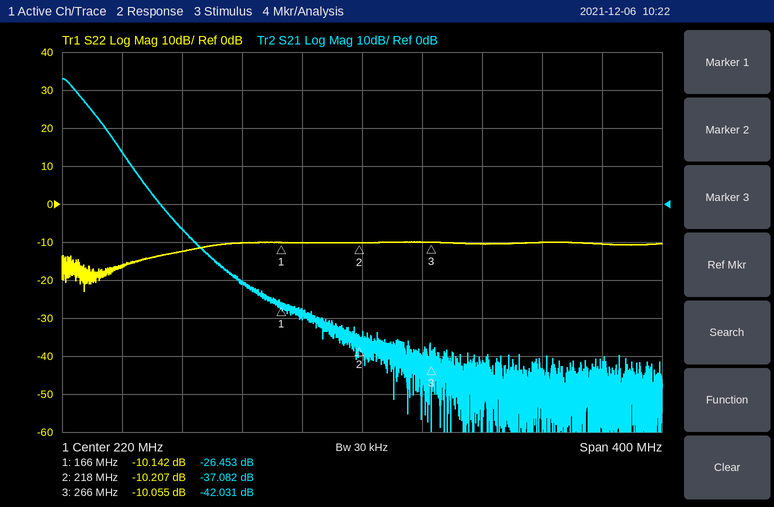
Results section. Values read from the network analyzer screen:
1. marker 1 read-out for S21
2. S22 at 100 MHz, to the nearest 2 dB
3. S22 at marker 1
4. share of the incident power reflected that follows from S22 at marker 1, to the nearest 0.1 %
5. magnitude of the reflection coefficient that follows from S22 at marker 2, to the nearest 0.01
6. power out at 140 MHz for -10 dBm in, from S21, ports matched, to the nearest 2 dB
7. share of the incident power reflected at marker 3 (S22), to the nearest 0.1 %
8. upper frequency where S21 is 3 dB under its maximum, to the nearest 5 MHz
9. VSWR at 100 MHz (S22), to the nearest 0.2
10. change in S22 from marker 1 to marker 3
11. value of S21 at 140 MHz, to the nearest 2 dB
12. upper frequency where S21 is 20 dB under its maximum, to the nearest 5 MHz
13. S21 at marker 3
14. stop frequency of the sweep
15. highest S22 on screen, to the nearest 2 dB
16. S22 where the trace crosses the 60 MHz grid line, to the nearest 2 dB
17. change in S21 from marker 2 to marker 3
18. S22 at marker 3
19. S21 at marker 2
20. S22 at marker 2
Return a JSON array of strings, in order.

["-26.453 dB", "-12 dB", "-10.142 dB", "9.7 %", "0.31", "-30 dBm", "9.9 %", "30 MHz", "1.6", "0.087 dB", "-20 dB", "60 MHz", "-42.031 dB", "420 MHz", "-10 dB", "-16 dB", "-4.949 dB", "-10.055 dB", "-37.082 dB", "-10.207 dB"]
